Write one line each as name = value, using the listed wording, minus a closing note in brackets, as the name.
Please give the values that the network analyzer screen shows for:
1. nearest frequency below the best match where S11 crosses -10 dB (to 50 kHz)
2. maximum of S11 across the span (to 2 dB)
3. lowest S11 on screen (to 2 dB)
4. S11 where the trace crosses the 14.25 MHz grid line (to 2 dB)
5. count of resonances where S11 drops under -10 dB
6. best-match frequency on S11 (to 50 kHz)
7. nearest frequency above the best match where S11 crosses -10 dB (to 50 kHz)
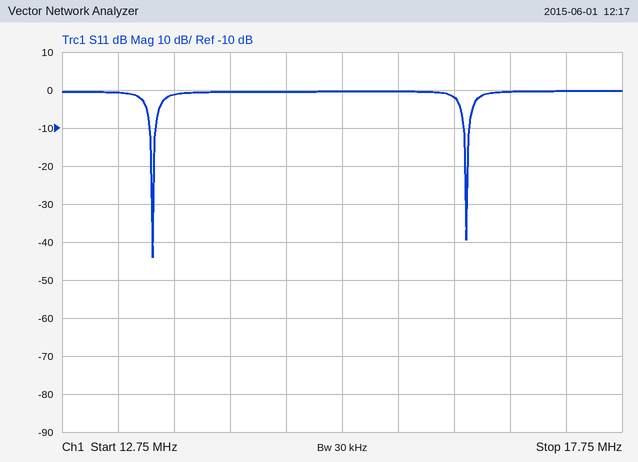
nearest frequency below the best match where S11 crosses -10 dB = 13.55 MHz
maximum of S11 across the span = 0 dB
lowest S11 on screen = -44 dB
S11 where the trace crosses the 14.25 MHz grid line = 0 dB
count of resonances where S11 drops under -10 dB = 2
best-match frequency on S11 = 13.55 MHz
nearest frequency above the best match where S11 crosses -10 dB = 13.60 MHz
